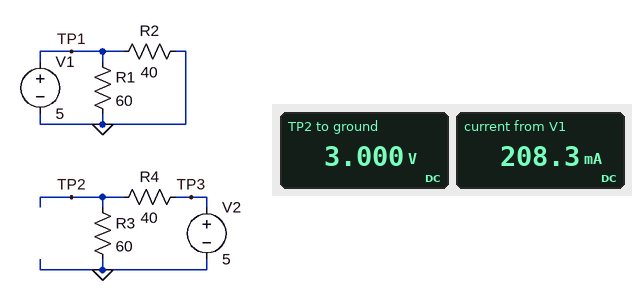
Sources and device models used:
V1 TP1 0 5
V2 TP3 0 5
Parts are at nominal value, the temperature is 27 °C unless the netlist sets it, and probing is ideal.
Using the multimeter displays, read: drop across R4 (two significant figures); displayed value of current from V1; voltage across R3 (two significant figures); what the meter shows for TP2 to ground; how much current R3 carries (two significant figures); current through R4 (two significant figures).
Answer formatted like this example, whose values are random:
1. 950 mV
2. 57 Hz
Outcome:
1. 2.0 V
2. 208.3 mA
3. 3.0 V
4. 3.000 V
5. 50 mA
6. 50 mA
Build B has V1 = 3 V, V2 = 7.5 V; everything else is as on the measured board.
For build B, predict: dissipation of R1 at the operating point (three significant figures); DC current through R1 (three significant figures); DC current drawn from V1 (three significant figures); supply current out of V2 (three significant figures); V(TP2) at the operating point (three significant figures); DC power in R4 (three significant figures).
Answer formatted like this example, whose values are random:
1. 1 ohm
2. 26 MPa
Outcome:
1. 150 mW
2. 50.0 mA
3. 125 mA
4. 75.0 mA
5. 4.50 V
6. 225 mW
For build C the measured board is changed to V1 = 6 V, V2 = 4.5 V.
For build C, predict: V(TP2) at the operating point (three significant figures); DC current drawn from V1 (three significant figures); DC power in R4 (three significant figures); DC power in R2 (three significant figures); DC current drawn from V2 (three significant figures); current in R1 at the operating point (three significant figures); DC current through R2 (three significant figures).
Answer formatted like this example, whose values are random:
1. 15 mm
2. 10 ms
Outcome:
1. 2.70 V
2. 250 mA
3. 81.0 mW
4. 900 mW
5. 45.0 mA
6. 100 mA
7. 150 mA
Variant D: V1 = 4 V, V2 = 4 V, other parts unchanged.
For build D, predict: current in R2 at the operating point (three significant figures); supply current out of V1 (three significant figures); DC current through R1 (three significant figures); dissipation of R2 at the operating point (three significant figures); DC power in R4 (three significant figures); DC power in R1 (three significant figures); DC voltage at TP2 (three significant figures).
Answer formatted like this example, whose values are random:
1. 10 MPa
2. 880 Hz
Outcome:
1. 100 mA
2. 167 mA
3. 66.7 mA
4. 400 mW
5. 64.0 mW
6. 267 mW
7. 2.40 V
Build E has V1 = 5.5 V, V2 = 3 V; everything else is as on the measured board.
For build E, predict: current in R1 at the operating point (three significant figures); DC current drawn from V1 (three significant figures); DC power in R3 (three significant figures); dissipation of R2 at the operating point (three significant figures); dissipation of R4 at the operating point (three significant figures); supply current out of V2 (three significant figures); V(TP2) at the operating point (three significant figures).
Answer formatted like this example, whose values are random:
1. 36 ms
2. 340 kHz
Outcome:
1. 91.7 mA
2. 229 mA
3. 54.0 mW
4. 756 mW
5. 36.0 mW
6. 30.0 mA
7. 1.80 V
